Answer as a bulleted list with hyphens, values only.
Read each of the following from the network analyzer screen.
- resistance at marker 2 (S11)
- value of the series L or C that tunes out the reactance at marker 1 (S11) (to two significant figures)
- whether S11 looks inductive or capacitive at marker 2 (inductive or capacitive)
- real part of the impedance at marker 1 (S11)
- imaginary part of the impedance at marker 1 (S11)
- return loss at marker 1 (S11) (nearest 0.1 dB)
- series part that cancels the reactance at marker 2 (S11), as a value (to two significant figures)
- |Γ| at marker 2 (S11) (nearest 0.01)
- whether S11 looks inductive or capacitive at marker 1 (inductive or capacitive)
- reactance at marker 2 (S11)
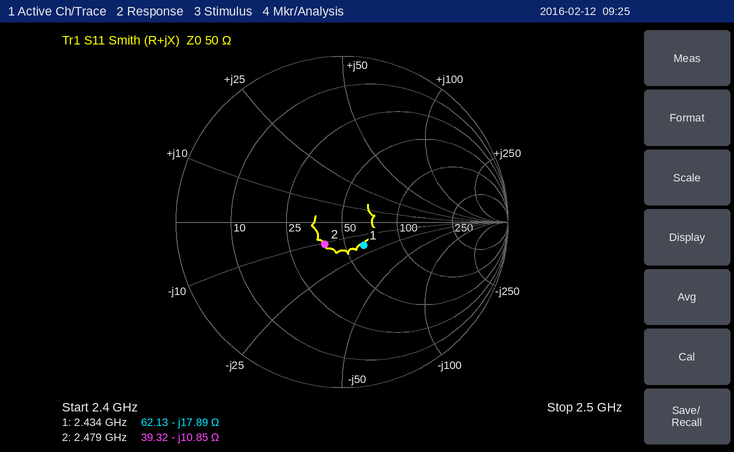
- 39.32 Ω
- 1.2 nH
- capacitive
- 62.13 Ω
- -17.89 Ω
- 14.4 dB
- 700 pH
- 0.17
- capacitive
- -10.85 Ω
